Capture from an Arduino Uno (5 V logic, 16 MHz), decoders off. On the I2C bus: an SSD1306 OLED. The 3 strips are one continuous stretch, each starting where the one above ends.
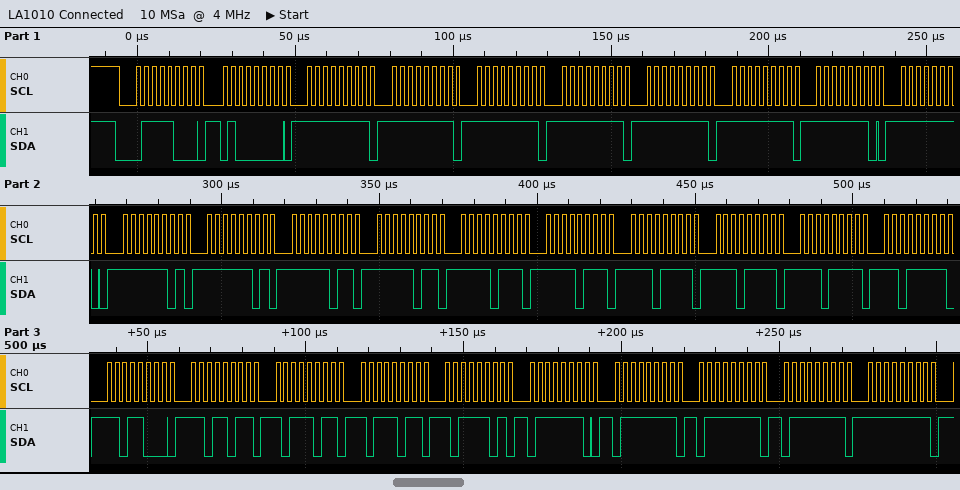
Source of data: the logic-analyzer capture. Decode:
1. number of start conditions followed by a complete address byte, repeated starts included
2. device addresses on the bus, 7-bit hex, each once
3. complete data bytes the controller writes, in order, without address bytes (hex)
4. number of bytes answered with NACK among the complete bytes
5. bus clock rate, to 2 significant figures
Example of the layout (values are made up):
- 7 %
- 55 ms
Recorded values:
- 1
- 0x3C
- 40 FF FF FF FF FF FF FE FE FD FD FB FB F7 F7 EF EF EF DF D8 DB BB BB BD 7E 7F 7F 7F FF
- 0
- 400 kHz
